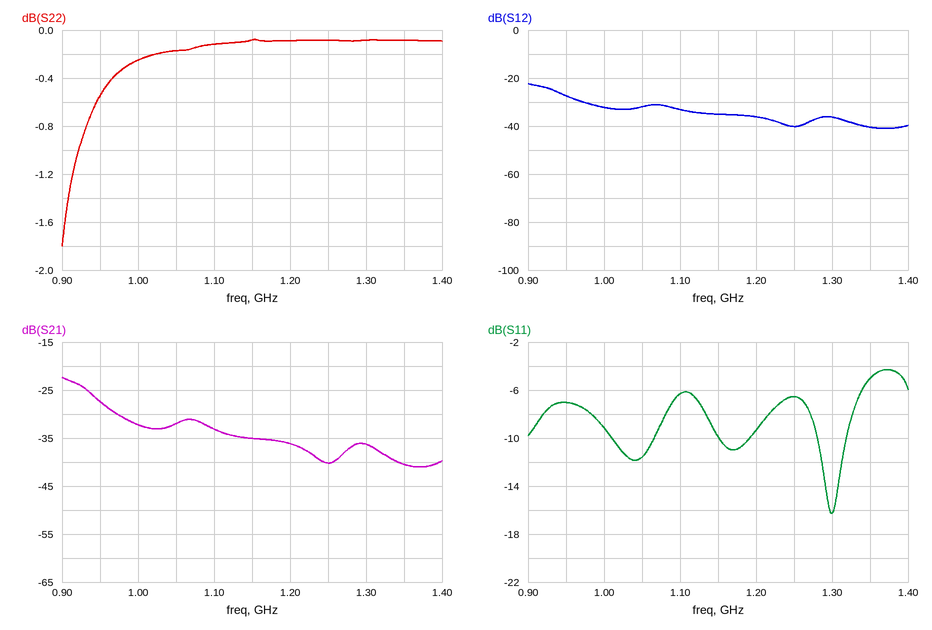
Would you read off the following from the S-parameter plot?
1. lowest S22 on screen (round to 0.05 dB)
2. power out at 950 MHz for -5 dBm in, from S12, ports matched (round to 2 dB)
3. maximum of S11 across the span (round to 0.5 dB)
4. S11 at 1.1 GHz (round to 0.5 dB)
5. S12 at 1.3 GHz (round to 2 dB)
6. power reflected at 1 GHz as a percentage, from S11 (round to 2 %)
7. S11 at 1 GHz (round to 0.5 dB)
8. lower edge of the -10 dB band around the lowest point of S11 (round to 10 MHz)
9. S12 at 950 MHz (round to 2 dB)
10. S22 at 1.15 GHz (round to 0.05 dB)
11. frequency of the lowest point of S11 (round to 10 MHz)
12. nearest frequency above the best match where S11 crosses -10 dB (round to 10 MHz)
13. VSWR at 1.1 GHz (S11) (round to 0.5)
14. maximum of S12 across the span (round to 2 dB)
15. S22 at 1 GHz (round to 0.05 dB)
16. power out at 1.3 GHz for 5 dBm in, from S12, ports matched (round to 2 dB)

-1.80 dB
-32 dBm
-4.5 dB
-6.5 dB
-36 dB
12 %
-9.0 dB
1.28 GHz
-28 dB
-0.10 dB
1.30 GHz
1.32 GHz
3.0
-22 dB
-0.25 dB
-32 dBm
